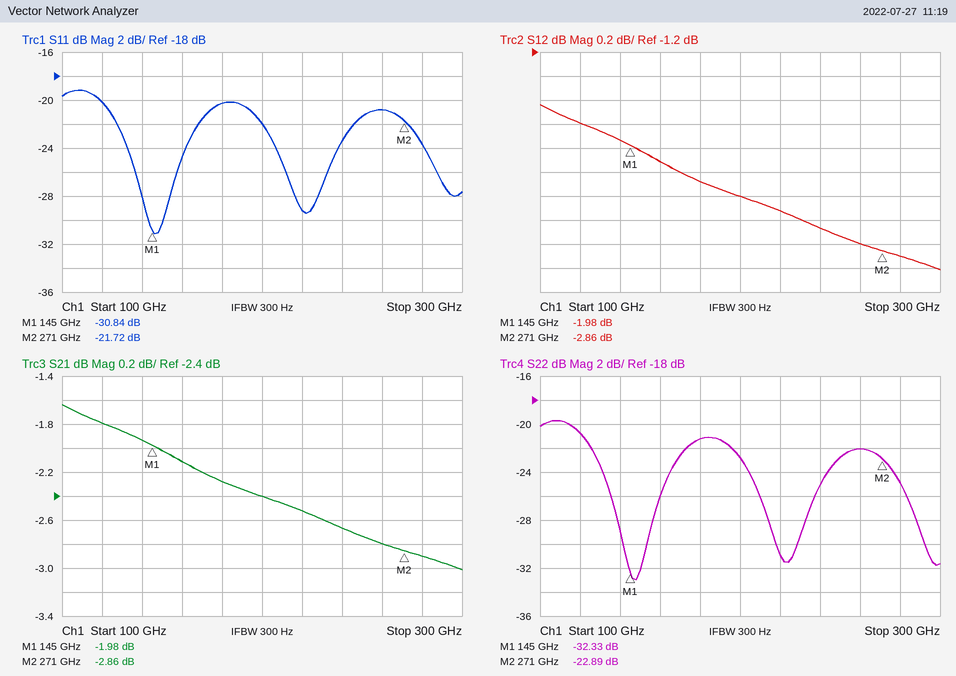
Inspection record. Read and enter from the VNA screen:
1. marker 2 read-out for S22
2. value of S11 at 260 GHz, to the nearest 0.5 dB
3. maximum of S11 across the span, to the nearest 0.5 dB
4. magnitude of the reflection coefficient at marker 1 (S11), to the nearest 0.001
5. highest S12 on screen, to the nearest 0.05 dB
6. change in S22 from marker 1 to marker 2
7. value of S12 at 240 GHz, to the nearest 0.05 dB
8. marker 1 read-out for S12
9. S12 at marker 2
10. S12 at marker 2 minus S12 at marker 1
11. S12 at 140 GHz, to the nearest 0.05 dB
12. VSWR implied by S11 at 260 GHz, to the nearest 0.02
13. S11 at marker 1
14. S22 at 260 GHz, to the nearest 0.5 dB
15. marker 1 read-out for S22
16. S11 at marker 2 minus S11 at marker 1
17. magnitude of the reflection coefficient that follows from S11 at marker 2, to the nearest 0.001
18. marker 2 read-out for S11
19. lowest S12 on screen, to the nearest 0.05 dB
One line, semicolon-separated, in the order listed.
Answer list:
-22.89 dB; -21.0 dB; -19.0 dB; 0.029; -1.65 dB; 9.44 dB; -2.65 dB; -1.98 dB; -2.86 dB; -0.88 dB; -1.95 dB; 1.20; -30.84 dB; -22.0 dB; -32.33 dB; 9.12 dB; 0.082; -21.72 dB; -3.00 dB
